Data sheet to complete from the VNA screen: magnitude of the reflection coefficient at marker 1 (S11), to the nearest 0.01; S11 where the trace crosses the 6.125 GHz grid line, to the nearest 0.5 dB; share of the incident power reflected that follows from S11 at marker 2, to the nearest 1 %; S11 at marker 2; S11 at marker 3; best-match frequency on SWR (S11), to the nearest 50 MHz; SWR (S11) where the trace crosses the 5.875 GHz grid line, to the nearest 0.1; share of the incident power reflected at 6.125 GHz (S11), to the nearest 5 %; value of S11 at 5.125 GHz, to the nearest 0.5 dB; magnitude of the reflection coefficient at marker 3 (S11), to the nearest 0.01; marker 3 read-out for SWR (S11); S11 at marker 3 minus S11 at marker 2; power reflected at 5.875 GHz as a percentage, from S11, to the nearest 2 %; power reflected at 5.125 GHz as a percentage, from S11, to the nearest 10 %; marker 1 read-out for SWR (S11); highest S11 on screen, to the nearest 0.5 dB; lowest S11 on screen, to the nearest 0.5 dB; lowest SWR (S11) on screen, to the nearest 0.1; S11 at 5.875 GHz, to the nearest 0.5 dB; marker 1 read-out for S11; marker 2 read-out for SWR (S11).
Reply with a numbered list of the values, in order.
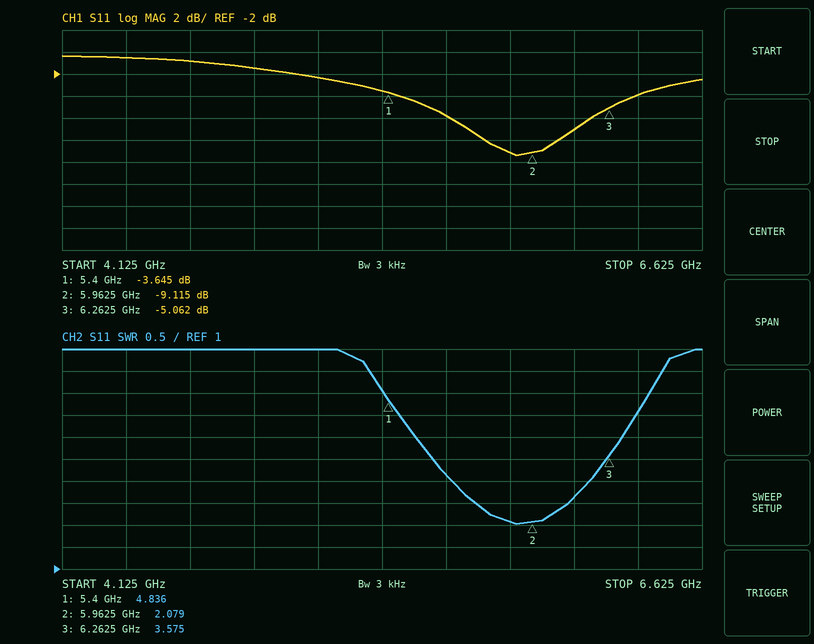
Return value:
1. 0.66
2. -7.0 dB
3. 12 %
4. -9.115 dB
5. -5.062 dB
6. 5.90 GHz
7. 2.1
8. 20 %
9. -2.5 dB
10. 0.56
11. 3.575
12. 4.053 dB
13. 12 %
14. 60 %
15. 4.836
16. -0.5 dB
17. -9.5 dB
18. 2.0
19. -9.0 dB
20. -3.645 dB
21. 2.079
